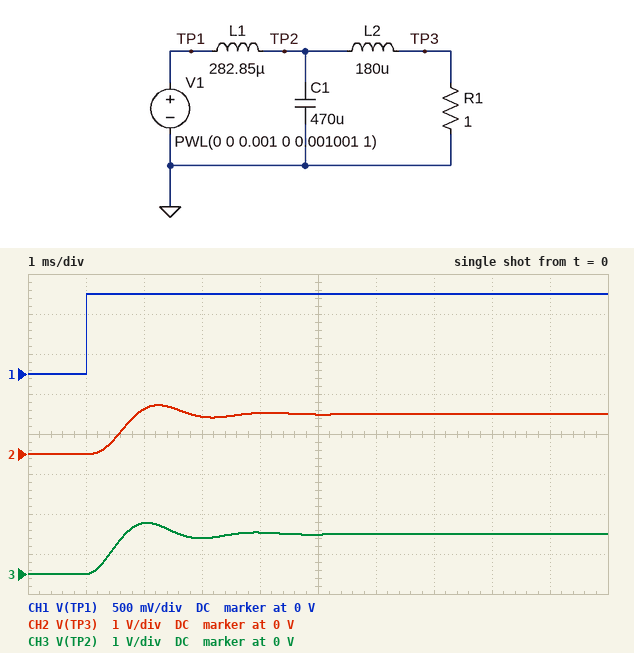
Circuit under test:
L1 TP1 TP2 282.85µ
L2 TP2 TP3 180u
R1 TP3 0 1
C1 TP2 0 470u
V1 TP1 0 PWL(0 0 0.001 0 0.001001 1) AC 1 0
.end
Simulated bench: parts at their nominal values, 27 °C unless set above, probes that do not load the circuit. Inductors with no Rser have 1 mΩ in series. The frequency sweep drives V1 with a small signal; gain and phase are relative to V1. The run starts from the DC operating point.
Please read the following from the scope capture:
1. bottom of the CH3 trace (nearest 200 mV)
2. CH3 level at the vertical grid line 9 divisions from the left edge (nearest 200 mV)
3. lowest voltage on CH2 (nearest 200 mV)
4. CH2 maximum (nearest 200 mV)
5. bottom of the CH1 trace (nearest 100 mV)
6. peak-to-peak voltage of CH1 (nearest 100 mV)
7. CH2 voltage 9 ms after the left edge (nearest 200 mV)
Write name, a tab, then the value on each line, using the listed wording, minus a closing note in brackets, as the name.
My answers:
bottom of the CH3 trace	0 V
CH3 level at the vertical grid line 9 divisions from the left edge	1.0 V
lowest voltage on CH2	0 V
CH2 maximum	1.2 V
bottom of the CH1 trace	0 V
peak-to-peak voltage of CH1	1.0 V
CH2 voltage 9 ms after the left edge	1.0 V
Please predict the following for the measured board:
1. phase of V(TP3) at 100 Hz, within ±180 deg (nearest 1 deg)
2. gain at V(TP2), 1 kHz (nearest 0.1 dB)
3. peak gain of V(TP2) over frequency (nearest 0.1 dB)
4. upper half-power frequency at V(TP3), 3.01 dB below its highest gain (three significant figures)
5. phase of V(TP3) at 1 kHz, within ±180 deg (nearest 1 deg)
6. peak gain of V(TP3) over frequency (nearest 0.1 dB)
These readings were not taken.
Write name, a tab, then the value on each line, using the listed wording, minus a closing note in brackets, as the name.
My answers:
phase of V(TP3) at 100 Hz, within ±180 deg	-17 deg
gain at V(TP2), 1 kHz	-10.8 dB
peak gain of V(TP2) over frequency	3.4 dB
upper half-power frequency at V(TP3), 3.01 dB below its highest gain	619 Hz
phase of V(TP3) at 1 kHz, within ±180 deg	145 deg
peak gain of V(TP3) over frequency	2.3 dB
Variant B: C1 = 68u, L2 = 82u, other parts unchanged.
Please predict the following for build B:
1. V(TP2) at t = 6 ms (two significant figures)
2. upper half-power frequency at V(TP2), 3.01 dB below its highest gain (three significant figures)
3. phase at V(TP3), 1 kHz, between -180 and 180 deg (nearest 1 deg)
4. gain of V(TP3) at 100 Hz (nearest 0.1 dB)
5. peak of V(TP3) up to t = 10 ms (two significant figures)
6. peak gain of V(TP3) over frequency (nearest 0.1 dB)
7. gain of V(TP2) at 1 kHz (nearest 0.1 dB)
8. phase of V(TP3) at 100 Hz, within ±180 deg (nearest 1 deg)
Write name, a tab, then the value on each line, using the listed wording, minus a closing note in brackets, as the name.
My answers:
V(TP2) at t = 6 ms	1.0 V
upper half-power frequency at V(TP2), 3.01 dB below its highest gain	601 Hz
phase at V(TP3), 1 kHz, between -180 and 180 deg	-83 deg
gain of V(TP3) at 100 Hz	-0.2 dB
peak of V(TP3) up to t = 10 ms	1.0 V
peak gain of V(TP3) over frequency	0 dB
gain of V(TP2) at 1 kHz	-4.6 dB
phase of V(TP3) at 100 Hz, within ±180 deg	-13 deg
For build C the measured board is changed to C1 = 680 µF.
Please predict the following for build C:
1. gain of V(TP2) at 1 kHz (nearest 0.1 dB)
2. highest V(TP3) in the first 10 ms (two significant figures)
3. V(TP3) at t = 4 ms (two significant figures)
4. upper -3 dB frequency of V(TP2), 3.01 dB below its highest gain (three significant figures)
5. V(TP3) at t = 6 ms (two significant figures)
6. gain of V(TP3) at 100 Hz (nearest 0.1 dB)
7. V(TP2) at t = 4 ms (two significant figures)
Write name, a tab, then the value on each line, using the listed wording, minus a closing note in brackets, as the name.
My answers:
gain of V(TP2) at 1 kHz	-15.2 dB
highest V(TP3) in the first 10 ms	1.3 V
V(TP3) at t = 4 ms	910 mV
upper -3 dB frequency of V(TP2), 3.01 dB below its highest gain	496 Hz
V(TP3) at t = 6 ms	980 mV
gain of V(TP3) at 100 Hz	0.3 dB
V(TP2) at t = 4 ms	940 mV
